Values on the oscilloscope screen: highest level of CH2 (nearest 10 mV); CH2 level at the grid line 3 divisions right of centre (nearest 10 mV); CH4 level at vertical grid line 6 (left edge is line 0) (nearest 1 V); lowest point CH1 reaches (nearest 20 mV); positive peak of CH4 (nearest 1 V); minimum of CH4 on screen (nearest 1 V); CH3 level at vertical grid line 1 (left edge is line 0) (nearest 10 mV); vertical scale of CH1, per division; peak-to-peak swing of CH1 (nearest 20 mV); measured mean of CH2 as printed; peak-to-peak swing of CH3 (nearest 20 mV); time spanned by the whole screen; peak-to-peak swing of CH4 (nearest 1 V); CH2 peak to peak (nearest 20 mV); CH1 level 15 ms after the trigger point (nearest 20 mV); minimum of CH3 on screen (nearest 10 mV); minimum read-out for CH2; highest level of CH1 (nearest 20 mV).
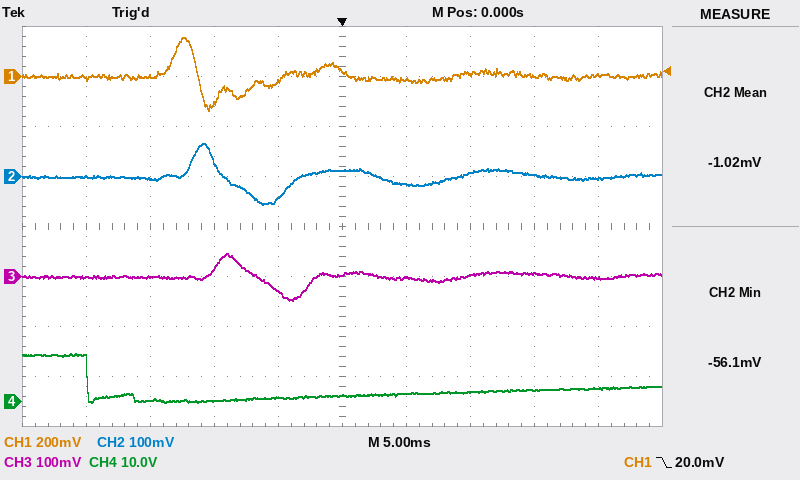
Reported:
70 mV
0 mV
2 V
-140 mV
10 V
0 V
0 mV
200 mV
300 mV
-1.02 mV
100 mV
50 ms
10 V
120 mV
0 mV
-50 mV
-56.1 mV
160 mV
